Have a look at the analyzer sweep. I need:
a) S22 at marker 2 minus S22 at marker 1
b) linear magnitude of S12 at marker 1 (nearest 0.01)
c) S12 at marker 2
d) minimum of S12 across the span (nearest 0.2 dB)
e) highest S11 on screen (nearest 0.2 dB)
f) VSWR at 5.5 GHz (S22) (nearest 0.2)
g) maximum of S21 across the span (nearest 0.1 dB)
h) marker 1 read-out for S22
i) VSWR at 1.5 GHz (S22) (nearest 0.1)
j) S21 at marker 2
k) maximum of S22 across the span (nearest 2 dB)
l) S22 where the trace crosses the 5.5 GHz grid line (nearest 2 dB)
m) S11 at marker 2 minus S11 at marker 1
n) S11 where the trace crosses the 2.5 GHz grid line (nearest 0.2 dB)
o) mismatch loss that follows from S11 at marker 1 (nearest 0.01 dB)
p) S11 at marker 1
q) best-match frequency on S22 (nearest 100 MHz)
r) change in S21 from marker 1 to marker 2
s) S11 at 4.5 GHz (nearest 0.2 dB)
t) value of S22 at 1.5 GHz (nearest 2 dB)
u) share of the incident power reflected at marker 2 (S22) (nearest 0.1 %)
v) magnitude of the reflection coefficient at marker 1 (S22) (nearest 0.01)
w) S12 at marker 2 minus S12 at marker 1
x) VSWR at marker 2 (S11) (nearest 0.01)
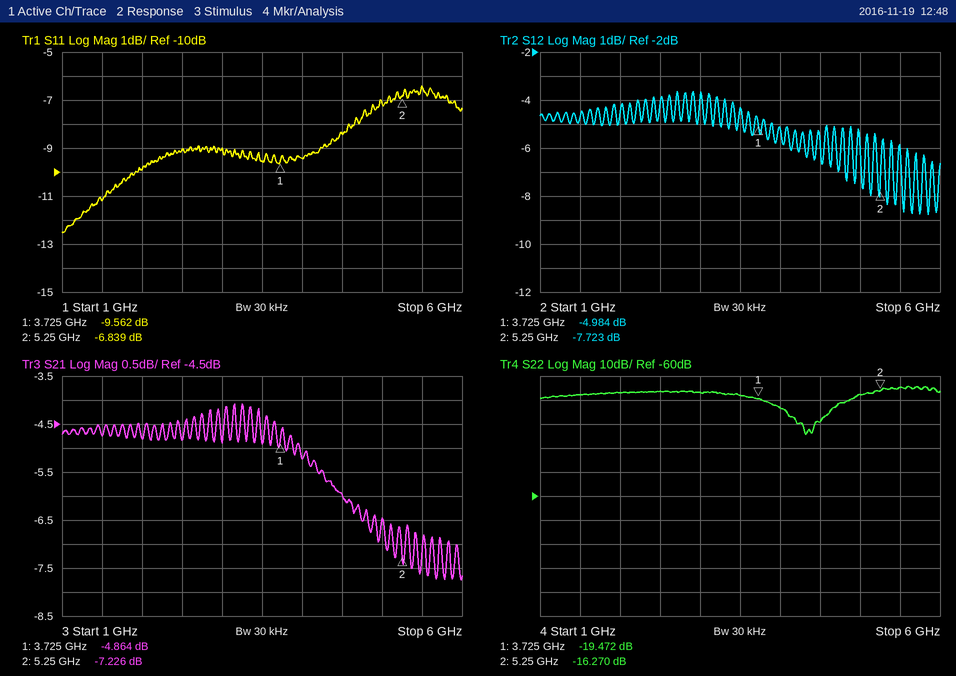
3.202 dB
0.56
-7.723 dB
-8.8 dB
-6.4 dB
1.4
-4.1 dB
-19.472 dB
1.3
-7.226 dB
-14 dB
-14 dB
2.723 dB
-9.0 dB
0.51 dB
-9.562 dB
4.3 GHz
-2.362 dB
-8.4 dB
-18 dB
2.4 %
0.11
-2.739 dB
2.67
